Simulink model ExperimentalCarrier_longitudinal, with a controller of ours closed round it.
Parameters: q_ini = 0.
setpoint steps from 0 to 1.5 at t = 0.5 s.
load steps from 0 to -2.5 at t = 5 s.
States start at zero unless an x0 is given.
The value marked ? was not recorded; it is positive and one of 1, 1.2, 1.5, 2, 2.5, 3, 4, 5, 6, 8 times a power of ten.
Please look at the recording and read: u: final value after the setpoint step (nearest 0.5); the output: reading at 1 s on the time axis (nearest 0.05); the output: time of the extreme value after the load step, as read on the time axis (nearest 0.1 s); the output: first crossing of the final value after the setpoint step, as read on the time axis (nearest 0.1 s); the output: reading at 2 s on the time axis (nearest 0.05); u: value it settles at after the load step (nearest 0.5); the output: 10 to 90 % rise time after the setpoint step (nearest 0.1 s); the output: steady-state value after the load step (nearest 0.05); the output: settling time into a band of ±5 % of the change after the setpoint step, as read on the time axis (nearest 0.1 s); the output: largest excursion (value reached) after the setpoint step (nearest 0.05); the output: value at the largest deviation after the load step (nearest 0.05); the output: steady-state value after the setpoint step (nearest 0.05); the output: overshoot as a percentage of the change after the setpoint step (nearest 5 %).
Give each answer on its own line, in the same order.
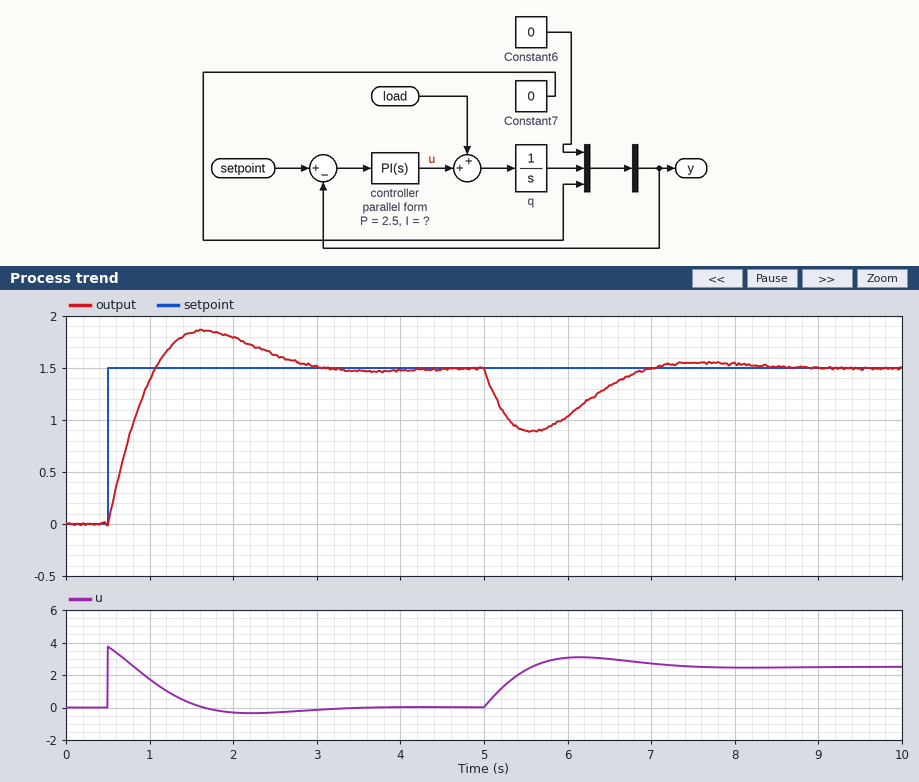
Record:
0.0
1.40
5.6 s
1.1 s
1.80
2.5
0.4 s
1.50
2.7 s
1.85
0.90
1.50
25 %
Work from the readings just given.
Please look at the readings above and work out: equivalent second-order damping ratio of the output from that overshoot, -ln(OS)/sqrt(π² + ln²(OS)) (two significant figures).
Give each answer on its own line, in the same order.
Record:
0.40
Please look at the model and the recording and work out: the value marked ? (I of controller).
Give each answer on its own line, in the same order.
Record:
4
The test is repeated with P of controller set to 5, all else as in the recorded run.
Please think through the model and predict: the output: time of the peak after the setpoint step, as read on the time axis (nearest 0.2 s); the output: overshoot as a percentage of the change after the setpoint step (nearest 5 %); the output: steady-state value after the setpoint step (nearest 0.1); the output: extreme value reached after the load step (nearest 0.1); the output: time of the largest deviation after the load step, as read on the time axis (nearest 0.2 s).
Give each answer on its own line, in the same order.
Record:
1.4 s
10 %
1.5
1.1
5.4 s
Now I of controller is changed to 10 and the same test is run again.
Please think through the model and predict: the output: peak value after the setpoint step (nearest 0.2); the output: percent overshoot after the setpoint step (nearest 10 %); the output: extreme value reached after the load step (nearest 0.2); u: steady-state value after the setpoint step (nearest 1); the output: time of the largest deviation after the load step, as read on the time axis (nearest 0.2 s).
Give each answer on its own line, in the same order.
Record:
2.0
40 %
1.0
0
5.4 s
